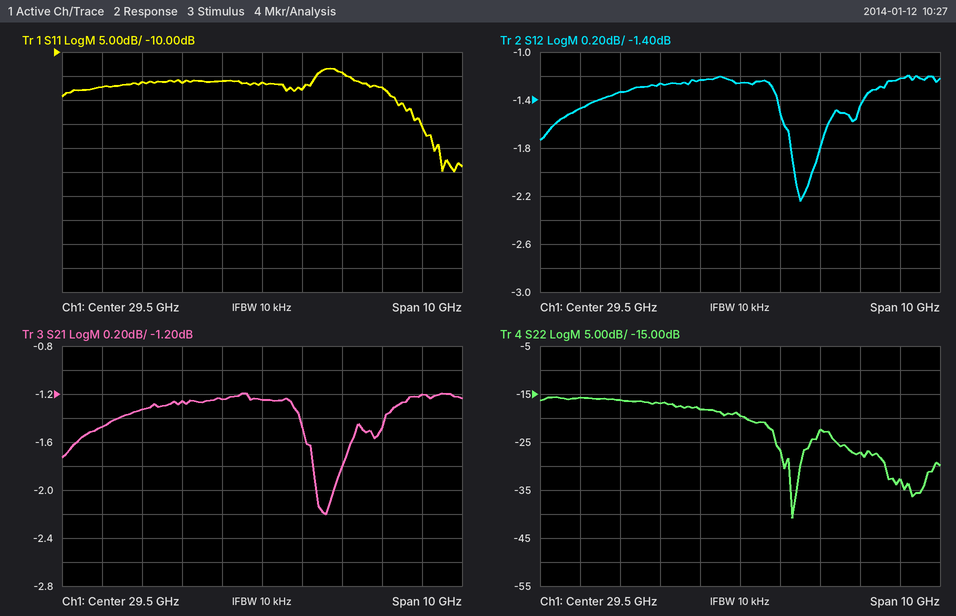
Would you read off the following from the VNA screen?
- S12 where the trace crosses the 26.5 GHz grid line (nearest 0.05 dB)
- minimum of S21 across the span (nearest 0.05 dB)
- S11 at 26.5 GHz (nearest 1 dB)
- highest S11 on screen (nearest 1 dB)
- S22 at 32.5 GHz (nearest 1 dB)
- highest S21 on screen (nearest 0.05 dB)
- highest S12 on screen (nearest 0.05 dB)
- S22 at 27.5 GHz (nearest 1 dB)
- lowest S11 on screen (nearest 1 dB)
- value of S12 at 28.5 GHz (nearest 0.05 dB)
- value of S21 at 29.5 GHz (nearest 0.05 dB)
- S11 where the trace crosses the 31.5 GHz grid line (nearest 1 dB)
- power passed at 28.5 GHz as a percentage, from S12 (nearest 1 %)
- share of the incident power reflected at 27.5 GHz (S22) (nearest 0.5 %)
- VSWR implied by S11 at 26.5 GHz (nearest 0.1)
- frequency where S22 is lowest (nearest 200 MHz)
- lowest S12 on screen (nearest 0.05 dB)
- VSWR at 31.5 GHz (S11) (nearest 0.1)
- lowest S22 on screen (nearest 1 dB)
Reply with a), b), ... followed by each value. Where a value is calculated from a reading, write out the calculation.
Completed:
a) -1.35 dB
b) -2.20 dB
c) -16 dB
d) -13 dB
e) -27 dB
f) -1.20 dB
g) -1.20 dB
h) -17 dB
i) -35 dB
j) -1.25 dB
k) -1.25 dB
l) -14 dB
m) 10^(-1.25/10) ≈ 75 %
n) 10^(-17/10) ≈ 2.0 %
o) |Γ| = 10^(-16/20) = 0.1585; VSWR = (1 + 0.1585)/(1 − 0.1585) ≈ 1.4
p) 30.8 GHz
q) -2.25 dB
r) |Γ| = 10^(-14/20) = 0.1995; VSWR = (1 + 0.1995)/(1 − 0.1995) ≈ 1.5
s) -41 dB
